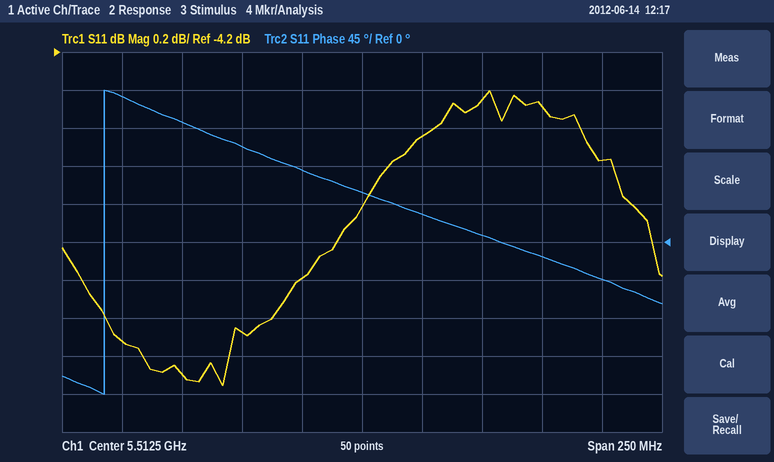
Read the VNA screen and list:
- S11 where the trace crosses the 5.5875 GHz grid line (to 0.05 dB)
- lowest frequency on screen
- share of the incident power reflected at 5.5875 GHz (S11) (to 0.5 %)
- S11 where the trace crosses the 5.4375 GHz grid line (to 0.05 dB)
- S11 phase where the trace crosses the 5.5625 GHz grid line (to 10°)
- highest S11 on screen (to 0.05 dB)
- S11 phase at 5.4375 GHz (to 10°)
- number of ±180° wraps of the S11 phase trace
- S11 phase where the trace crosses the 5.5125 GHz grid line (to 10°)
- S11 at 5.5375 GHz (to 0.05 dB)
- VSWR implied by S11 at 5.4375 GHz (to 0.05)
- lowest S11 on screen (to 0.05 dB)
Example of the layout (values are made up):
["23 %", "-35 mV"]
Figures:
["-4.50 dB", "5.3875 GHz", "35.5 %", "-5.90 dB", "10°", "-4.40 dB", "140°", "1", "60°", "-4.65 dB", "3.05", "-5.95 dB"]
